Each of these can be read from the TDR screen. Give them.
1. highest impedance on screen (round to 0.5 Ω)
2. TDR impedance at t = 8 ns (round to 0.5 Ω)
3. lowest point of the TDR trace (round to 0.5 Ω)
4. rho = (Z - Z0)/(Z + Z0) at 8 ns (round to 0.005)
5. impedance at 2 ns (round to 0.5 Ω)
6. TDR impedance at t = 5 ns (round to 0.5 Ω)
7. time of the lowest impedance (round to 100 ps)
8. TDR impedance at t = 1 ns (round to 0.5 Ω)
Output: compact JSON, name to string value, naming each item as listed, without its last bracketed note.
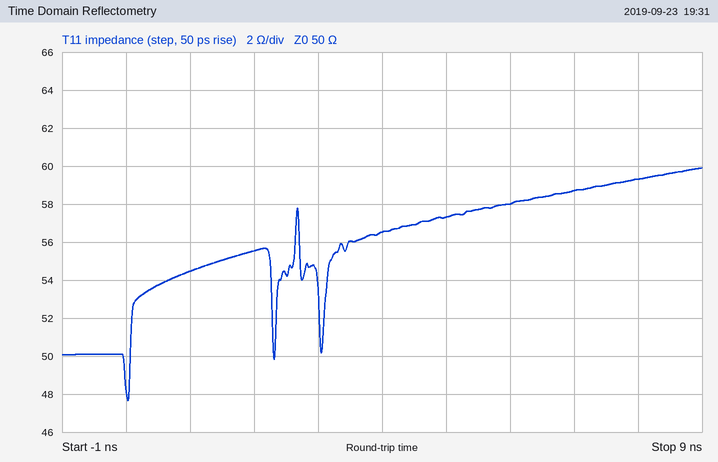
{"highest impedance on screen": "60.0 Ω", "TDR impedance at t = 8 ns": "59.5 Ω", "lowest point of the TDR trace": "47.5 Ω", "rho = (Z - Z0)/(Z + Z0) at 8 ns": "+0.085", "impedance at 2 ns": "55.5 Ω", "TDR impedance at t = 5 ns": "57.5 Ω", "time of the lowest impedance": "0.0 ns", "TDR impedance at t = 1 ns": "54.5 Ω"}
